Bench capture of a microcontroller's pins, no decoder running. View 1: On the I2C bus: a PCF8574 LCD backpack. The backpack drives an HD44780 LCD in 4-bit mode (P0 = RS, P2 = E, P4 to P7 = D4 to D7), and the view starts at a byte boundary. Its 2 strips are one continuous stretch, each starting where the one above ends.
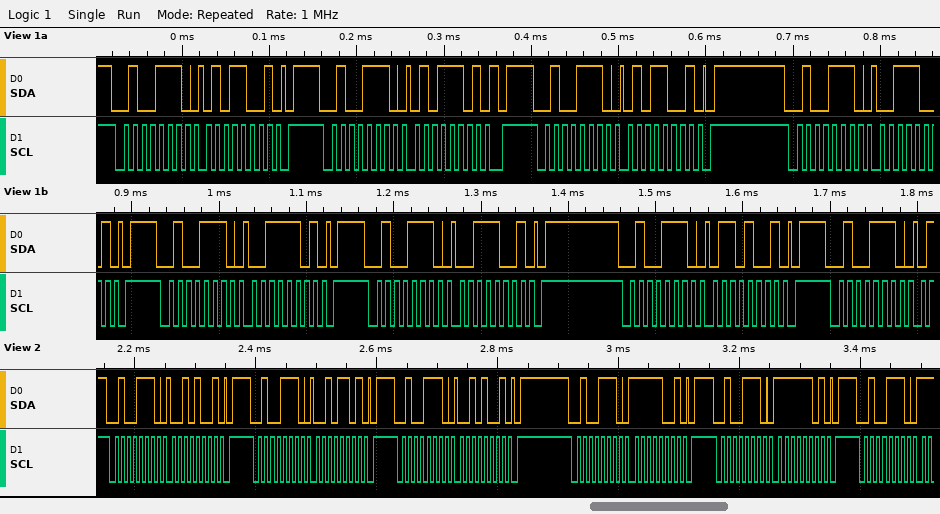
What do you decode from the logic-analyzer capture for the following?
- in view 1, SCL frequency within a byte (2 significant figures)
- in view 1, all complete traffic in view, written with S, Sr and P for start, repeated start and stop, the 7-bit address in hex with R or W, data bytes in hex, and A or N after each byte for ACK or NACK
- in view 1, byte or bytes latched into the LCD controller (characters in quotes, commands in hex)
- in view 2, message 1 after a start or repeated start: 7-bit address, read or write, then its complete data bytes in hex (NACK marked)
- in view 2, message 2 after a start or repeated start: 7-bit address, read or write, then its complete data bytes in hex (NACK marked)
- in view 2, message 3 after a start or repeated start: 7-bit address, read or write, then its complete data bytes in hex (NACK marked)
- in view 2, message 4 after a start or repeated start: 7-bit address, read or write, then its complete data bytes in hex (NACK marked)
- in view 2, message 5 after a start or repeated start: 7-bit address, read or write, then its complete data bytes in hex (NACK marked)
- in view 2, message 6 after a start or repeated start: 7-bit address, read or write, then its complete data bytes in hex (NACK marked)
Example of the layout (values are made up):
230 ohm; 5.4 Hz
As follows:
100 kHz; S 27W A 59 A P S 27W A 5D A P S 27W A 59 A P S 27W A 39 A P S 27W A 3D A P S 27W A 39 A P S 27W A 69 A P S 27W A; 'S'; 0x27 write: 29; 0x27 write: 2D; 0x27 write: 29; 0x27 write: F9; 0x27 write: FD; 0x27 write
